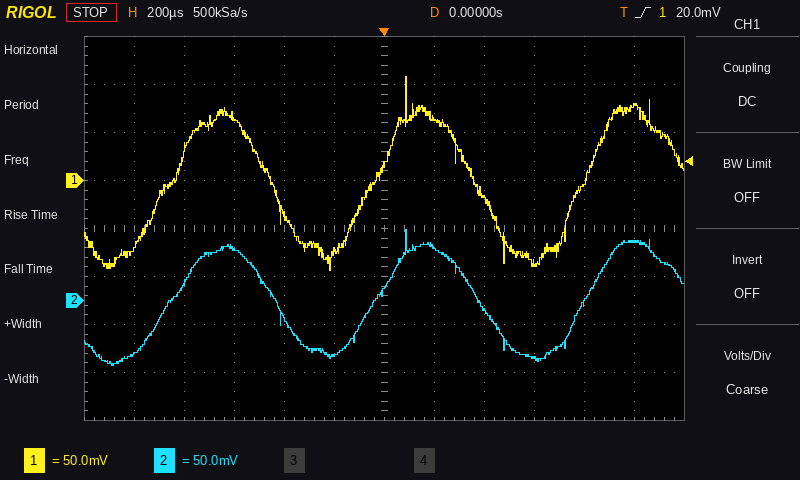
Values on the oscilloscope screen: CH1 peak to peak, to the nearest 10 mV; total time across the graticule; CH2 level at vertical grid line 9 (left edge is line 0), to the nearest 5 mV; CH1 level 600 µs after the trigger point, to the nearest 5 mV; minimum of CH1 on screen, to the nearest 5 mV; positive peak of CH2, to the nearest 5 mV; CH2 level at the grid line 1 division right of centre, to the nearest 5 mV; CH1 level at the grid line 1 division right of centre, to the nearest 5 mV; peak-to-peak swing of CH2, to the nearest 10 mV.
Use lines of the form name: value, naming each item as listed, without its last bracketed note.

CH1 peak to peak, to the nearest 10 mV: 200 mV
total time across the graticule: 2.4 ms
CH2 level at vertical grid line 9 (left edge is line 0), to the nearest 5 mV: -60 mV
CH1 level 600 µs after the trigger point, to the nearest 5 mV: -85 mV
minimum of CH1 on screen, to the nearest 5 mV: -95 mV
positive peak of CH2, to the nearest 5 mV: 75 mV
CH2 level at the grid line 1 division right of centre, to the nearest 5 mV: 55 mV
CH1 level at the grid line 1 division right of centre, to the nearest 5 mV: 65 mV
peak-to-peak swing of CH2, to the nearest 10 mV: 140 mV
